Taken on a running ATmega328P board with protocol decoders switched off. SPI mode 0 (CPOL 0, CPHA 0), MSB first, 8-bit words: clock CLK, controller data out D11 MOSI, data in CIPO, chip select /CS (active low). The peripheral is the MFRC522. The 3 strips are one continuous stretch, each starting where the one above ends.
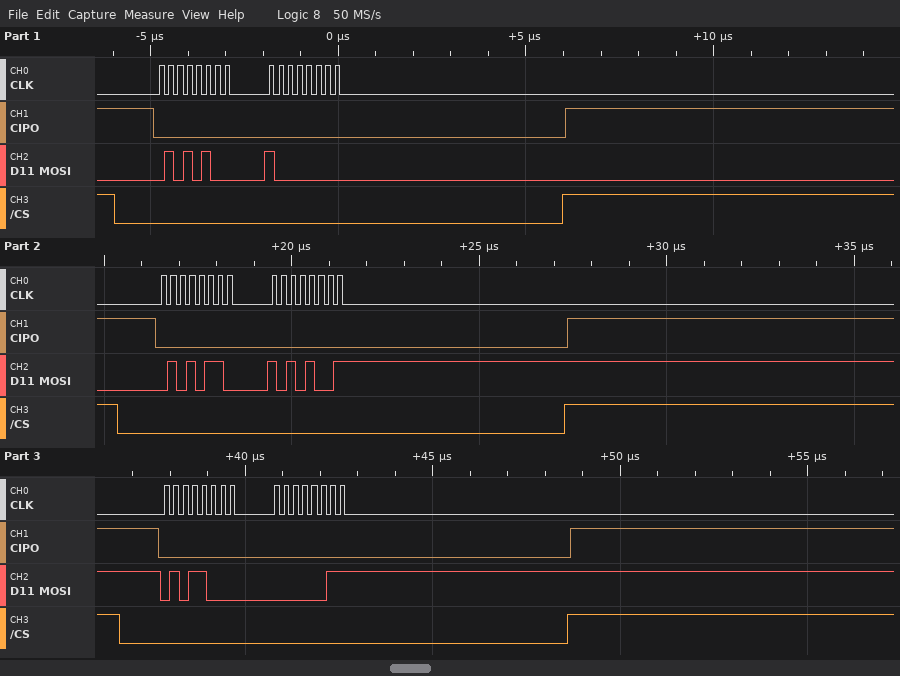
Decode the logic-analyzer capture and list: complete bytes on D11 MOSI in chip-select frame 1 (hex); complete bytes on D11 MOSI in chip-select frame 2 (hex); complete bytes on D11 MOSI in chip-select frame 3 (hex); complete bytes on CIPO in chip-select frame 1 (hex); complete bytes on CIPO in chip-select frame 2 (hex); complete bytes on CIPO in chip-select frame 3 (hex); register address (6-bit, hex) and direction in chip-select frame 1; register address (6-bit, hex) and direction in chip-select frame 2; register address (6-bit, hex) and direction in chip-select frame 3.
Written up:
0x54 0x80
0x56 0xA9
0x58 0x03
0x00 0x00
0x00 0x00
0x00 0x00
0x2A write
0x2B write
0x2C write
